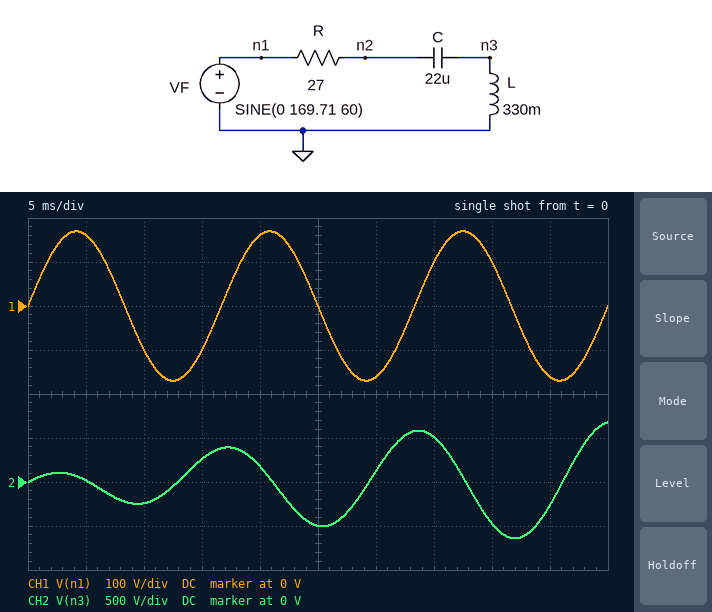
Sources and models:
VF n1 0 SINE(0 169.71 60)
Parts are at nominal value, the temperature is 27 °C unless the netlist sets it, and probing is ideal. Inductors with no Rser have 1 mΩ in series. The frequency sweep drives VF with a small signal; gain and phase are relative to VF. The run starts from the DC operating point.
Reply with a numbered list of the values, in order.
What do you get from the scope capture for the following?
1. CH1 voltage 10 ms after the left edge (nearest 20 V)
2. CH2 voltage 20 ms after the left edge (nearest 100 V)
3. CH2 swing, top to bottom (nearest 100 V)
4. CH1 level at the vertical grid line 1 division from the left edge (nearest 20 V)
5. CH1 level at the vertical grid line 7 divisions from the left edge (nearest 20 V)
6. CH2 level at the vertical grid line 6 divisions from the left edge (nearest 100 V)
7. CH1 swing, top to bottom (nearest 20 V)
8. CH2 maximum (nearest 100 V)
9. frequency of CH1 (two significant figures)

1. -100 V
2. 200 V
3. 1.3 kV
4. 160 V
5. 100 V
6. 100 V
7. 340 V
8. 700 V
9. 60 Hz
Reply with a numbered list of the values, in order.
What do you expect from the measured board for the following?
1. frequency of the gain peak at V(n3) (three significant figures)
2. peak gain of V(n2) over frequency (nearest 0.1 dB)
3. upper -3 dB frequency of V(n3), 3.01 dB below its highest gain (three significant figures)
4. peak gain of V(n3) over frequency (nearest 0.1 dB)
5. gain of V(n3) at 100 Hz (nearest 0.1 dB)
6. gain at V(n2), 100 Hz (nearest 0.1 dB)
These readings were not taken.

1. 59.8 Hz
2. 0 dB
3. 67.9 Hz
4. 13.2 dB
5. 3.6 dB
6. -0.2 dB
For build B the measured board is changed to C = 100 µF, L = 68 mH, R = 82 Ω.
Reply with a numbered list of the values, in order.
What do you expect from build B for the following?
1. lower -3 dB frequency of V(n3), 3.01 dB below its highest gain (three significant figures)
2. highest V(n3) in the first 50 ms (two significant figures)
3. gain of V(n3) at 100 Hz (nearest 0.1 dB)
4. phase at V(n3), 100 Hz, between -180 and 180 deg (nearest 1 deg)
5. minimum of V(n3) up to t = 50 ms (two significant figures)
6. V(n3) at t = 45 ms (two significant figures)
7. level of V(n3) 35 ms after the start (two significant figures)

1. 173 Hz
2. 54 V
3. -6.1 dB
4. 72 deg
5. -53 V
6. -16 V
7. 43 V
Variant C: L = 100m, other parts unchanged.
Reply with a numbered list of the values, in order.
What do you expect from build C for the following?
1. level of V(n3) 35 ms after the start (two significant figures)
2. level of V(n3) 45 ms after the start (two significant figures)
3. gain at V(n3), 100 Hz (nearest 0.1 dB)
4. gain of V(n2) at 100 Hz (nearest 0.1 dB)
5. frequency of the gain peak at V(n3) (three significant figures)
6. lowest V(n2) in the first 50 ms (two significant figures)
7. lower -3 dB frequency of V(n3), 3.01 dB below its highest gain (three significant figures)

1. -24 V
2. 59 V
3. 6.8 dB
4. -9.6 dB
5. 112 Hz
6. -170 V
7. 93.7 Hz
